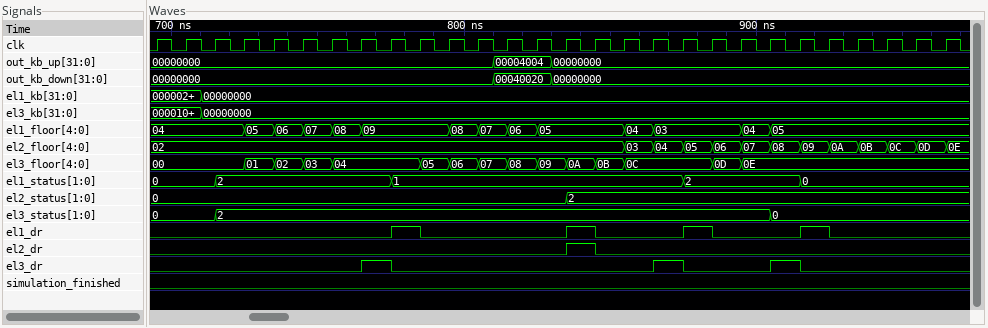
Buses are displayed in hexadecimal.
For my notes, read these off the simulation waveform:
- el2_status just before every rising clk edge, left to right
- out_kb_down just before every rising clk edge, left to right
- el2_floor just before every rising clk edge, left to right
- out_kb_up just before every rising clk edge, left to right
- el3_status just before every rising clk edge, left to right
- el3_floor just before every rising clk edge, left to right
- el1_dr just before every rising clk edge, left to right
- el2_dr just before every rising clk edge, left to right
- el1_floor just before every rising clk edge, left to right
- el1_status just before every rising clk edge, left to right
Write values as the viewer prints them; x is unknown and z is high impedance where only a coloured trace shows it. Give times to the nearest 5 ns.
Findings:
0, 0, 0, 0, 0, 0, 0, 0, 0, 0, 0, 0, 0, 0, 0, 2, 2, 2, 2, 2, 2, 2, 2, 2, 2, 2, 2, 2
00000000, 00000000, 00000000, 00000000, 00000000, 00000000, 00000000, 00000000, 00000000, 00000000, 00000000, 00000000, 00040020, 00040020, 00000000, 00000000, 00000000, 00000000, 00000000, 00000000, 00000000, 00000000, 00000000, 00000000, 00000000, 00000000, 00000000, 00000000
02, 02, 02, 02, 02, 02, 02, 02, 02, 02, 02, 02, 02, 02, 02, 02, 02, 03, 04, 05, 06, 07, 08, 09, 0A, 0B, 0C, 0D
00000000, 00000000, 00000000, 00000000, 00000000, 00000000, 00000000, 00000000, 00000000, 00000000, 00000000, 00000000, 00004004, 00004004, 00000000, 00000000, 00000000, 00000000, 00000000, 00000000, 00000000, 00000000, 00000000, 00000000, 00000000, 00000000, 00000000, 00000000
0, 0, 0, 2, 2, 2, 2, 2, 2, 2, 2, 2, 2, 2, 2, 2, 2, 2, 2, 2, 2, 2, 0, 0, 0, 0, 0, 0
00, 00, 00, 00, 01, 02, 03, 04, 04, 04, 05, 06, 07, 08, 09, 0A, 0B, 0C, 0C, 0C, 0D, 0E, 0E, 0E, 0E, 0E, 0E, 0E
0 0 0 0 0 0 0 0 0 1 0 0 0 0 0 1 0 0 0 1 0 0 0 1 0 0 0 0
0 0 0 0 0 0 0 0 0 0 0 0 0 0 0 1 0 0 0 0 0 0 0 0 0 0 0 0
04, 04, 04, 04, 05, 06, 07, 08, 09, 09, 09, 08, 07, 06, 05, 05, 05, 04, 03, 03, 03, 04, 05, 05, 05, 05, 05, 05
0, 0, 0, 2, 2, 2, 2, 2, 2, 1, 1, 1, 1, 1, 1, 1, 1, 1, 1, 2, 2, 2, 2, 0, 0, 0, 0, 0
